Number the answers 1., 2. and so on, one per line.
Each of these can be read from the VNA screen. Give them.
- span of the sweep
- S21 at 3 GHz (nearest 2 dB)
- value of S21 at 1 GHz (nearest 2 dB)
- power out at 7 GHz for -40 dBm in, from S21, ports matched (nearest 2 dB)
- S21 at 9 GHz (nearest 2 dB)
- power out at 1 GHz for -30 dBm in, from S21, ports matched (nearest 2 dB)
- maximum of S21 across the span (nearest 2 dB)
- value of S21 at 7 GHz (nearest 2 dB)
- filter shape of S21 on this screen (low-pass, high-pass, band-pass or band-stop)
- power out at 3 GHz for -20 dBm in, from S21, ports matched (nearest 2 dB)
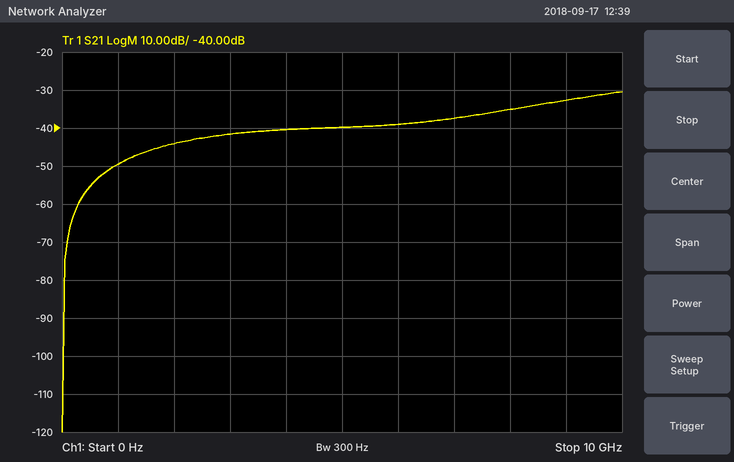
1. 10 GHz
2. -42 dB
3. -50 dB
4. -78 dBm
5. -32 dB
6. -80 dBm
7. -30 dB
8. -38 dB
9. high-pass
10. -62 dBm
